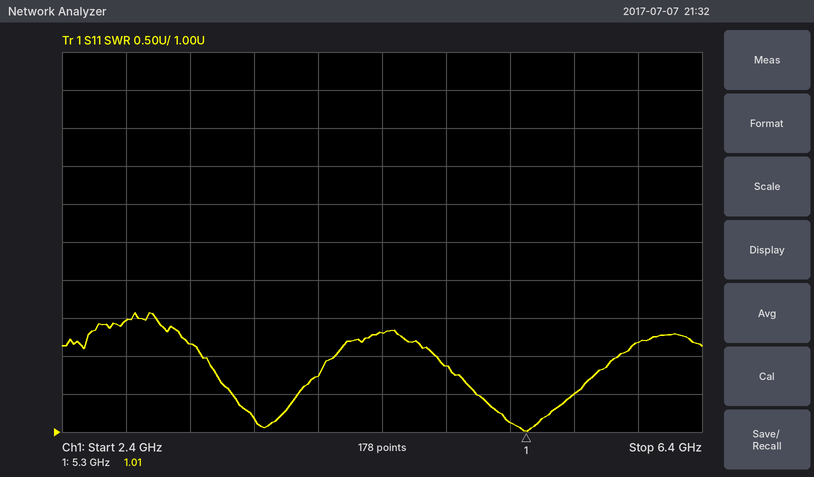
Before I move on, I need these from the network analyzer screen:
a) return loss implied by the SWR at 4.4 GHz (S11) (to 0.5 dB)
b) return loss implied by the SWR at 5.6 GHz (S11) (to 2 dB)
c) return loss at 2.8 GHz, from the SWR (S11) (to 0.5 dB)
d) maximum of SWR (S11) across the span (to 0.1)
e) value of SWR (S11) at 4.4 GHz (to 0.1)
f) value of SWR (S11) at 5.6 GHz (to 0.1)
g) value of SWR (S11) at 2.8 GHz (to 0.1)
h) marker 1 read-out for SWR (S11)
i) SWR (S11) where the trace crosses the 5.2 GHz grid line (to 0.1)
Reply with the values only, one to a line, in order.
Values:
8.0 dB
14 dB
7.5 dB
2.6
2.3
1.5
2.5
1.01
1.1
